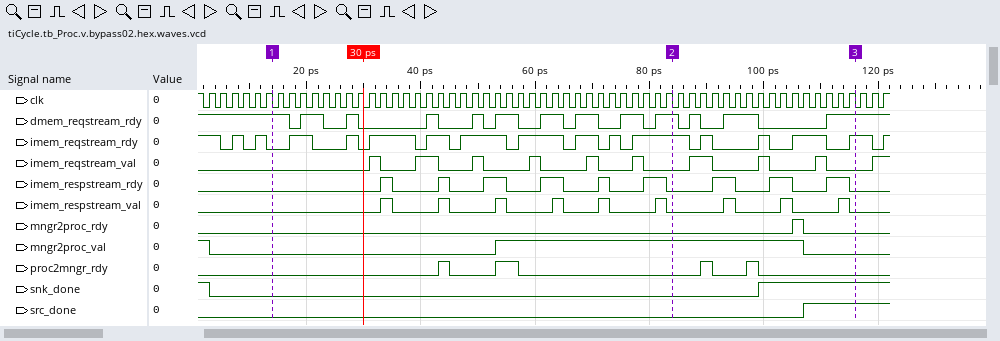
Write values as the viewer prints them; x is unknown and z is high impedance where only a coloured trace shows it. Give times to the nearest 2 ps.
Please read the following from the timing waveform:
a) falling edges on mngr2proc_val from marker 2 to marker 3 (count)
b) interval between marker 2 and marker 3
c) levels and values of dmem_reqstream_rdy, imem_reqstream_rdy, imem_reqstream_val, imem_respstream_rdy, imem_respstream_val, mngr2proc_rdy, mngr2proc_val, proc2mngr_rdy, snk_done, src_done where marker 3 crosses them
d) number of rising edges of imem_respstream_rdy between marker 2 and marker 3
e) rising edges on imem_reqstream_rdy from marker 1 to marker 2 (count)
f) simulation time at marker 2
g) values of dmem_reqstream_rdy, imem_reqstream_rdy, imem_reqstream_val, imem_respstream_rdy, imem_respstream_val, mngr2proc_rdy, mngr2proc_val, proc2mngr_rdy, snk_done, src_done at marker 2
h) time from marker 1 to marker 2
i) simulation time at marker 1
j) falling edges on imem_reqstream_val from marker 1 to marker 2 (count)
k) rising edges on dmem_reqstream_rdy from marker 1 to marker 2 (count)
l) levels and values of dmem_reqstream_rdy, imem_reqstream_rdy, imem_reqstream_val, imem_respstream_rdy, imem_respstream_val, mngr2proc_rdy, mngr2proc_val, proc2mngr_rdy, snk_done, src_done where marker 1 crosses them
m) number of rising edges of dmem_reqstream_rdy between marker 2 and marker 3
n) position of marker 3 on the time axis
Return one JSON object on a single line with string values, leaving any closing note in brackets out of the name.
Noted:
{"falling edges on mngr2proc_val from marker 2 to marker 3": "1", "interval between marker 2 and marker 3": "32 ps", "levels and values of dmem_reqstream_rdy, imem_reqstream_rdy, imem_reqstream_val, imem_respstream_rdy, imem_respstream_val, mngr2proc_rdy, mngr2proc_val, proc2mngr_rdy, snk_done, src_done where marker 3 crosses them": "dmem_reqstream_rdy=1, imem_reqstream_rdy=1, imem_reqstream_val=0, imem_respstream_rdy=0, imem_respstream_val=0, mngr2proc_rdy=0, mngr2proc_val=0, proc2mngr_rdy=0, snk_done=1, src_done=1", "number of rising edges of imem_respstream_rdy between marker 2 and marker 3": "3", "rising edges on imem_reqstream_rdy from marker 1 to marker 2": "9", "simulation time at marker 2": "84 ps", "values of dmem_reqstream_rdy, imem_reqstream_rdy, imem_reqstream_val, imem_respstream_rdy, imem_respstream_val, mngr2proc_rdy, mngr2proc_val, proc2mngr_rdy, snk_done, src_done at marker 2": "dmem_reqstream_rdy=1, imem_reqstream_rdy=1, imem_reqstream_val=0, imem_respstream_rdy=0, imem_respstream_val=0, mngr2proc_rdy=0, mngr2proc_val=1, proc2mngr_rdy=0, snk_done=0, src_done=0", "time from marker 1 to marker 2": "70 ps", "simulation time at marker 1": "14 ps", "falling edges on imem_reqstream_val from marker 1 to marker 2": "6", "rising edges on dmem_reqstream_rdy from marker 1 to marker 2": "9", "levels and values of dmem_reqstream_rdy, imem_reqstream_rdy, imem_reqstream_val, imem_respstream_rdy, imem_respstream_val, mngr2proc_rdy, mngr2proc_val, proc2mngr_rdy, snk_done, src_done where marker 1 crosses them": "dmem_reqstream_rdy=1, imem_reqstream_rdy=0, imem_reqstream_val=0, imem_respstream_rdy=0, imem_respstream_val=0, mngr2proc_rdy=0, mngr2proc_val=0, proc2mngr_rdy=0, snk_done=0, src_done=0", "number of rising edges of dmem_reqstream_rdy between marker 2 and marker 3": "3", "position of marker 3 on the time axis": "116 ps"}
